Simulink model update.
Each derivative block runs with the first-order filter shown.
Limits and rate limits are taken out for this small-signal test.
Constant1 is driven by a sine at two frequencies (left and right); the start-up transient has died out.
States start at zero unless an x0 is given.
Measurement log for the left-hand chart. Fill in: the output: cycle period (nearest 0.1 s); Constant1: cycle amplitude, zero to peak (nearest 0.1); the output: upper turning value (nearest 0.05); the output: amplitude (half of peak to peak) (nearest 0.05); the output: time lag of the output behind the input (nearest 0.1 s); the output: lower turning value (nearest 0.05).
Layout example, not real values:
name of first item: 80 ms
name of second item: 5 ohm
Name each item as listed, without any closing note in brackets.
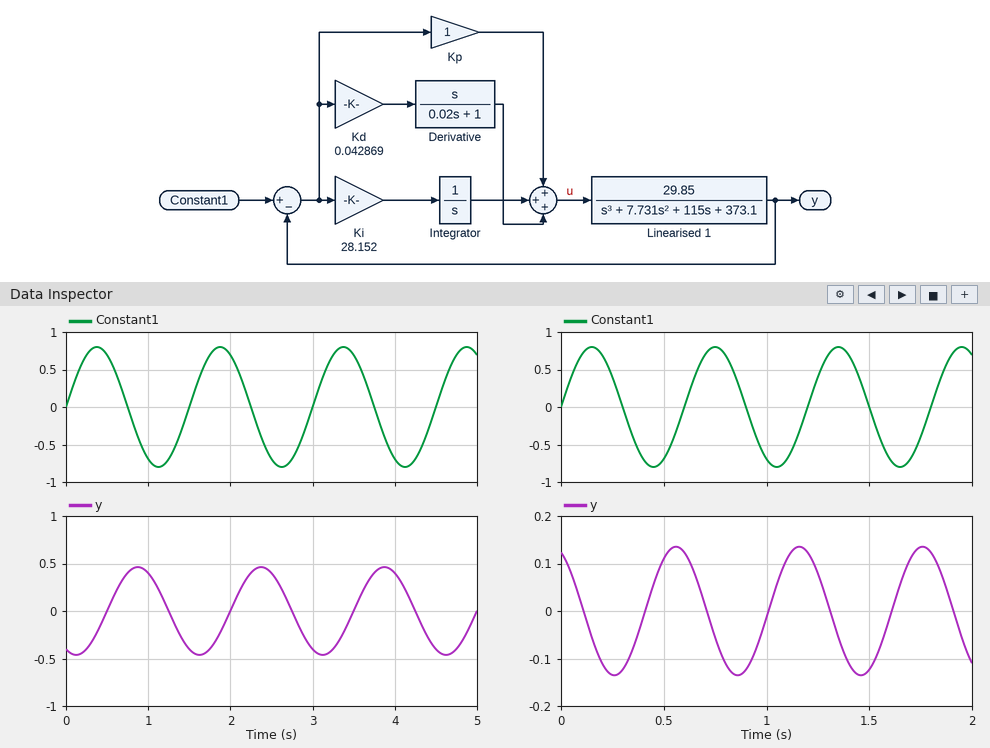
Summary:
the output: cycle period: 1.5 s
Constant1: cycle amplitude, zero to peak: 0.8
the output: upper turning value: 0.45
the output: amplitude (half of peak to peak): 0.45
the output: time lag of the output behind the input: 0.5 s
the output: lower turning value: -0.45
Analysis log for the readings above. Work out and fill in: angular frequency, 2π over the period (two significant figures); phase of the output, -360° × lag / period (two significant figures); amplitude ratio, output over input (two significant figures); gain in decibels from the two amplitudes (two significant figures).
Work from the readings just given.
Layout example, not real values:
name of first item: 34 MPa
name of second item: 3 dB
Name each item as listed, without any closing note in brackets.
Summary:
angular frequency, 2π over the period: 4.2 rad/s
phase of the output, -360° × lag / period: -120°
amplitude ratio, output over input: 0.56
gain in decibels from the two amplitudes: -5.0 dB
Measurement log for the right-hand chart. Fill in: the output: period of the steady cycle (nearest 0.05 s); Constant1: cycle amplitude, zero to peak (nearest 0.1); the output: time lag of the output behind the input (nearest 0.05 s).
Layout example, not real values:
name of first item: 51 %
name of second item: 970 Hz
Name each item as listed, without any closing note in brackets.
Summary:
the output: period of the steady cycle: 0.60 s
Constant1: cycle amplitude, zero to peak: 0.8
the output: time lag of the output behind the input: 0.40 s
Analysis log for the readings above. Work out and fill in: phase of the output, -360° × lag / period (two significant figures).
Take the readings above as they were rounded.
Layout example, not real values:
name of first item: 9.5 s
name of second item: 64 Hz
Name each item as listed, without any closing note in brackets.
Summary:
phase of the output, -360° × lag / period: -240°
